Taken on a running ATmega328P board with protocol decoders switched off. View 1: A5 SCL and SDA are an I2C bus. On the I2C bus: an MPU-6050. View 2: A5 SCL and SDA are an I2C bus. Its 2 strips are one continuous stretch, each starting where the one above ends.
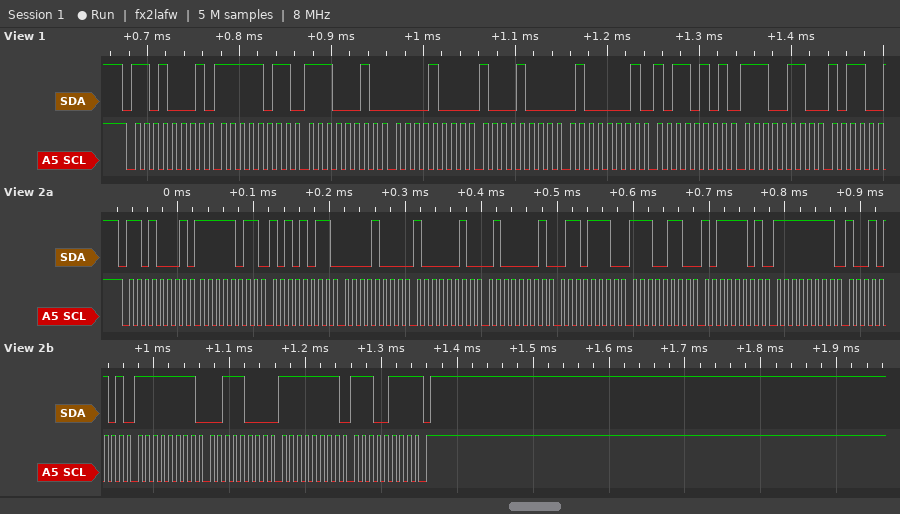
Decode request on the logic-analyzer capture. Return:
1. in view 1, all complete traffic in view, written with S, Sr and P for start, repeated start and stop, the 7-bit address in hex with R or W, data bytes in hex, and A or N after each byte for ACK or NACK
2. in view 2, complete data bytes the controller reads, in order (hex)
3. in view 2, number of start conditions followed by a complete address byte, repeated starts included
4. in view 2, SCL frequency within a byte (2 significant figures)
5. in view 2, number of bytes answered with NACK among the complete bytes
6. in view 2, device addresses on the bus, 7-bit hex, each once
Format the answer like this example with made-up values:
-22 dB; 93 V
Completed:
S 68R A FB A E2 A 08 A 88 A 41 A B5 A E6 A; FB AB 08 82 41 6E E6 BD FF 95 FF 38 FF E7; 1; 100 kHz; 1; 0x68
